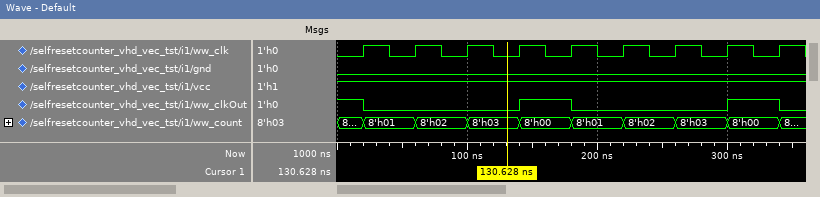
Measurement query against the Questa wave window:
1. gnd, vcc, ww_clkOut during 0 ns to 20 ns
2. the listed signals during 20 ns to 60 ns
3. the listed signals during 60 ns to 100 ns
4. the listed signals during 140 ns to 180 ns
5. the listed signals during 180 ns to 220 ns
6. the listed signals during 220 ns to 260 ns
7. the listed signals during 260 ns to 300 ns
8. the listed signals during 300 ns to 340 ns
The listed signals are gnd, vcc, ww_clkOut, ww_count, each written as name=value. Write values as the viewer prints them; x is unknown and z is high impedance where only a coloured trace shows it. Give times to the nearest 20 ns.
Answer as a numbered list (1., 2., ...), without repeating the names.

1. gnd=0, vcc=1, ww_clkOut=1
2. gnd=0, vcc=1, ww_clkOut=0, ww_count=8'h01
3. gnd=0, vcc=1, ww_clkOut=0, ww_count=8'h02
4. gnd=0, vcc=1, ww_clkOut=1, ww_count=8'h00
5. gnd=0, vcc=1, ww_clkOut=0, ww_count=8'h01
6. gnd=0, vcc=1, ww_clkOut=0, ww_count=8'h02
7. gnd=0, vcc=1, ww_clkOut=0, ww_count=8'h03
8. gnd=0, vcc=1, ww_clkOut=1, ww_count=8'h00
